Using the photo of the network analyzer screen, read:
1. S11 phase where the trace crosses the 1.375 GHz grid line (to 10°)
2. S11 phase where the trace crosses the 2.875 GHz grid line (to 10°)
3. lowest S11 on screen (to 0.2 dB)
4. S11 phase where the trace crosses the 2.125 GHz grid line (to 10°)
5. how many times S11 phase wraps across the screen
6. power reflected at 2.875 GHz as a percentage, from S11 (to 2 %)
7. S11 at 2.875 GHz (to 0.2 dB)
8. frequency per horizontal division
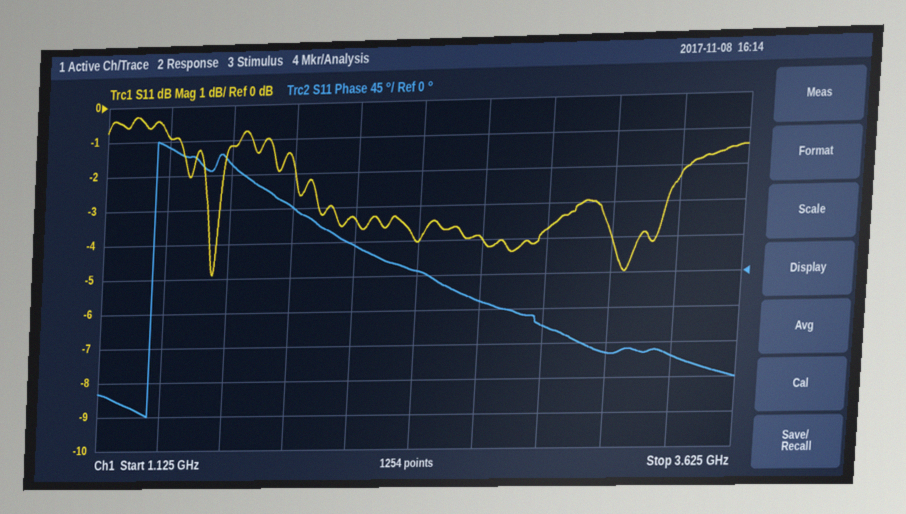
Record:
170°
-70°
-5.0 dB
40°
1
42 %
-3.8 dB
250 MHz
